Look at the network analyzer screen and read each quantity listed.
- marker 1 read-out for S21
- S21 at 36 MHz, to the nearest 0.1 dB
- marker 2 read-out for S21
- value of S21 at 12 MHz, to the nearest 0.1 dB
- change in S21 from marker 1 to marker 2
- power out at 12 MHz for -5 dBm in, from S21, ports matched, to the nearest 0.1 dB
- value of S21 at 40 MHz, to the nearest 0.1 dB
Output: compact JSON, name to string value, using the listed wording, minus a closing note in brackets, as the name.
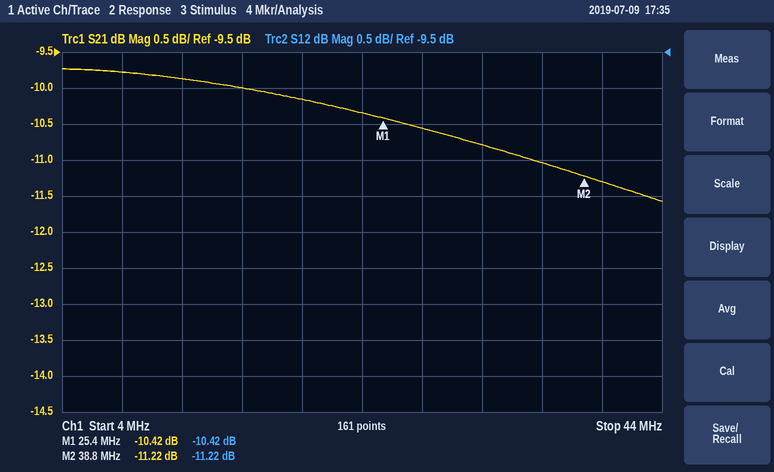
{"marker 1 read-out for S21": "-10.42 dB", "S21 at 36 MHz, to the nearest 0.1 dB": "-11.0 dB", "marker 2 read-out for S21": "-11.22 dB", "value of S21 at 12 MHz, to the nearest 0.1 dB": "-9.9 dB", "change in S21 from marker 1 to marker 2": "-0.80 dB", "power out at 12 MHz for -5 dBm in, from S21, ports matched, to the nearest 0.1 dB": "-14.9 dBm", "value of S21 at 40 MHz, to the nearest 0.1 dB": "-11.3 dB"}
